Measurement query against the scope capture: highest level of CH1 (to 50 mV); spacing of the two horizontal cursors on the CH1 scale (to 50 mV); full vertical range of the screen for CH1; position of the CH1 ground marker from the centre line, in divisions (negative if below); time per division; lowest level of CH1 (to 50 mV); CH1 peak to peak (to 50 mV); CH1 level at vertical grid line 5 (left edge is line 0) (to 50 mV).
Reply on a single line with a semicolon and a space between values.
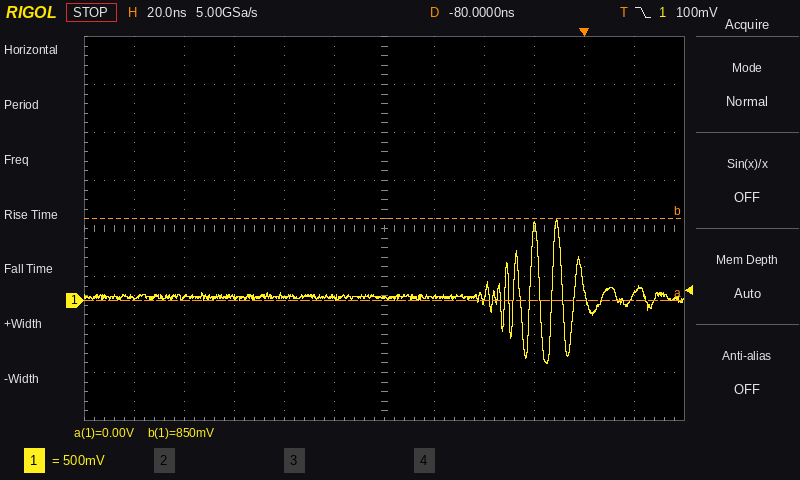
850 mV; 850 mV; 4 V; -1.5 div; 20 ns; -650 mV; 1.50 V; 50 mV
